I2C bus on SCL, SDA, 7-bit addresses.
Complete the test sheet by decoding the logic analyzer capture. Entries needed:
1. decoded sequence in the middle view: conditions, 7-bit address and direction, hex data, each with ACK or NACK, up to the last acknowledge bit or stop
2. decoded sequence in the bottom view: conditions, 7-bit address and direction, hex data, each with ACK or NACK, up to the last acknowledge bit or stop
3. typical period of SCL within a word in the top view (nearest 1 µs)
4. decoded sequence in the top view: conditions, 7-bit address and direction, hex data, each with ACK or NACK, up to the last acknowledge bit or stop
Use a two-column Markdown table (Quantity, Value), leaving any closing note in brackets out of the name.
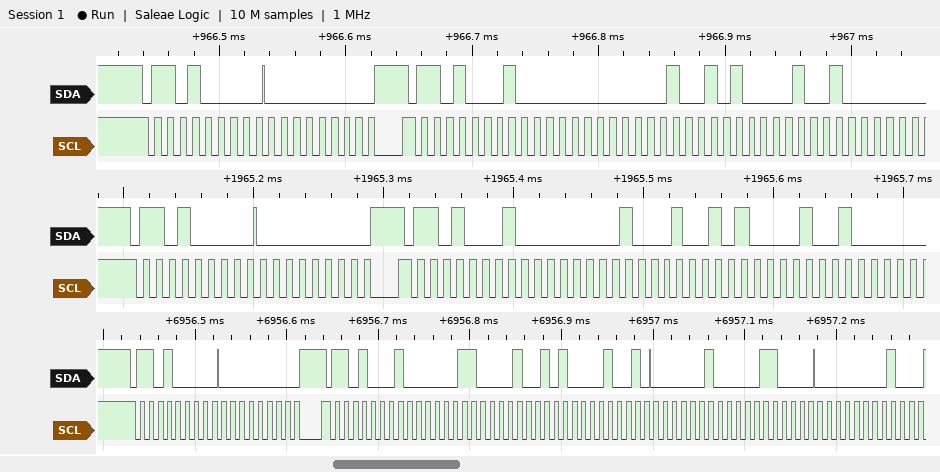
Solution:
| Quantity | Value |
|---|---|
| decoded sequence in the middle view: conditions, 7-bit address and direction, hex data, each with ACK or NACK, up to the last acknowledge bit or stop | start, address 68 write ACK, 00 ACK, repeated start, address 68 read ACK, 01 ACK, 25 ACK, 12 ACK |
| decoded sequence in the bottom view: conditions, 7-bit address and direction, hex data, each with ACK or NACK, up to the last acknowledge bit or stop | start, address 68 write ACK, 00 ACK, repeated start, address 68 read ACK, 06 ACK, 25 ACK, 12 ACK, 04 ACK, 30 ACK, 01 ACK |
| typical period of SCL within a word in the top view | 10 µs |
| decoded sequence in the top view: conditions, 7-bit address and direction, hex data, each with ACK or NACK, up to the last acknowledge bit or stop | start, address 68 write ACK, 00 ACK, repeated start, address 68 read ACK, 00 ACK, 25 ACK, 12 ACK |
